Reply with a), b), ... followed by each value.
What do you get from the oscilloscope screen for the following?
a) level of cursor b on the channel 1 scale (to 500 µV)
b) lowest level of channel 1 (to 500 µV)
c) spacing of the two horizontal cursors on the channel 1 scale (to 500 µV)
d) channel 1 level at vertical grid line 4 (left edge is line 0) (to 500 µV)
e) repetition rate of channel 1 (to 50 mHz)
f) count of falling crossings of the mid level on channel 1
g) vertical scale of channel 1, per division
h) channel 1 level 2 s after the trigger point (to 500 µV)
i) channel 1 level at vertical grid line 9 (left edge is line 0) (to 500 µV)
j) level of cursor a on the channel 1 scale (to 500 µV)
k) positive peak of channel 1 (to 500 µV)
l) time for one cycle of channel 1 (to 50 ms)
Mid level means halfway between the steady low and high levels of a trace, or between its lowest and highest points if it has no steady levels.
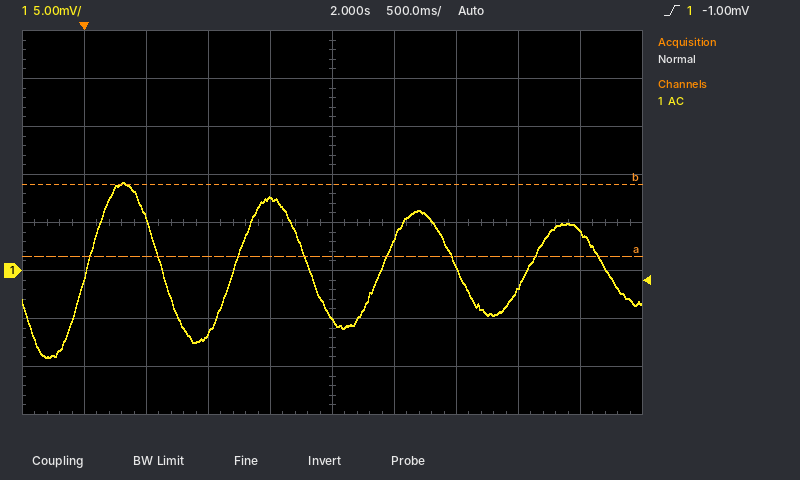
a) 9.0 mV
b) -9.0 mV
c) 7.5 mV
d) 7.5 mV
e) 850 mHz
f) 4
g) 5 mV
h) -5.0 mV
i) 4.0 mV
j) 1.5 mV
k) 9.0 mV
l) 1.20 s
